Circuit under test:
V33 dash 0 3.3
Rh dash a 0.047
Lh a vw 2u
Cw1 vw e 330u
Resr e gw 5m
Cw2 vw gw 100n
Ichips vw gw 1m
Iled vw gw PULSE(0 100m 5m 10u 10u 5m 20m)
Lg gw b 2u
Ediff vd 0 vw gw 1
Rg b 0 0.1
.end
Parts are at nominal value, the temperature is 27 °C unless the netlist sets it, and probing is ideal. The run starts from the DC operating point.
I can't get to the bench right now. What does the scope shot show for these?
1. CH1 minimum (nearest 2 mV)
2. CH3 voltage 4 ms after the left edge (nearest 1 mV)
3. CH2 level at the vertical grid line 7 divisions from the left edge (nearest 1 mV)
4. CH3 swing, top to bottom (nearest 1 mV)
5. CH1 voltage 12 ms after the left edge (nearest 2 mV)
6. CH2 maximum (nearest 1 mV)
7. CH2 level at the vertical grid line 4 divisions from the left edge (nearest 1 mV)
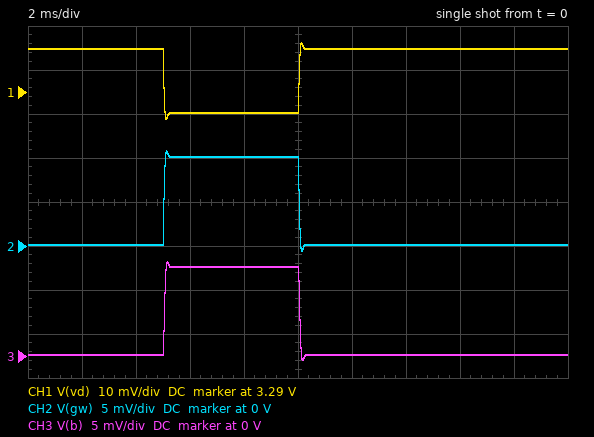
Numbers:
3.284 V
0 V
0 V
11 mV
3.300 V
11 mV
10 mV
